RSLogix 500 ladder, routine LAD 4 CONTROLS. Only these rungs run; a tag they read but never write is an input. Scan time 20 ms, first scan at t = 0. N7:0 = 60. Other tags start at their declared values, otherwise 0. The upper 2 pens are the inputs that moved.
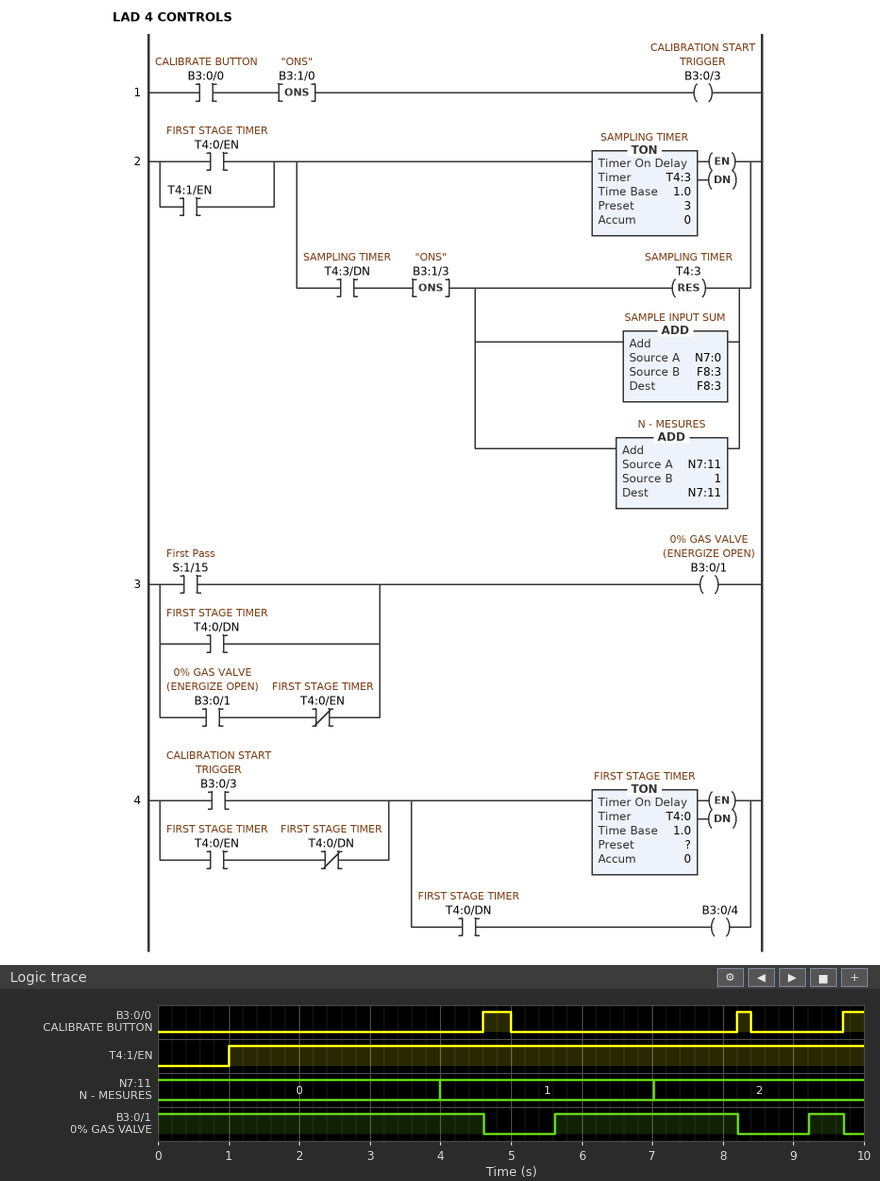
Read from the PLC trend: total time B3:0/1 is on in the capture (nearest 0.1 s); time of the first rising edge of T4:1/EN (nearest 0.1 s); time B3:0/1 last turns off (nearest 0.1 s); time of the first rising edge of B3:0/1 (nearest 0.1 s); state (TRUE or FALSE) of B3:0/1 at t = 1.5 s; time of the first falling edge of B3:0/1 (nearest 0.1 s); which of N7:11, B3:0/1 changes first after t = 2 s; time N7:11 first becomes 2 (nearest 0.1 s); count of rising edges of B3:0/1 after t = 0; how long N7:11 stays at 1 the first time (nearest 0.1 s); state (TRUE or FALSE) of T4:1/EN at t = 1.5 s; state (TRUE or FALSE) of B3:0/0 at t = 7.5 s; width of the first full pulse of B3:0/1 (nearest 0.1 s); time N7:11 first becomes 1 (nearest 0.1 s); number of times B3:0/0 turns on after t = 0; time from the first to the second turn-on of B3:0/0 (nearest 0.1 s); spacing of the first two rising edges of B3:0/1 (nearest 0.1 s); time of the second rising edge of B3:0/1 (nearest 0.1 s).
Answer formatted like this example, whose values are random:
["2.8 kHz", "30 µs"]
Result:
["7.7 s", "1.0 s", "9.7 s", "5.6 s", "TRUE", "4.6 s", "N7:11", "7.0 s", "2", "3.0 s", "TRUE", "FALSE", "2.6 s", "4.0 s", "3", "3.6 s", "3.6 s", "9.2 s"]
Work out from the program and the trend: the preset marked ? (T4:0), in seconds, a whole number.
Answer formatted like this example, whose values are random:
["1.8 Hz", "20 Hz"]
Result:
["1 s"]
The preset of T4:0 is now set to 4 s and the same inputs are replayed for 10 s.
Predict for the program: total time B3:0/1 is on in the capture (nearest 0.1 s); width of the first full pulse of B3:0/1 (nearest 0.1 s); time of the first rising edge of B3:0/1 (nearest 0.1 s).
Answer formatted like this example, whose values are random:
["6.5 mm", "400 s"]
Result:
["5.7 s", "1.1 s", "8.6 s"]
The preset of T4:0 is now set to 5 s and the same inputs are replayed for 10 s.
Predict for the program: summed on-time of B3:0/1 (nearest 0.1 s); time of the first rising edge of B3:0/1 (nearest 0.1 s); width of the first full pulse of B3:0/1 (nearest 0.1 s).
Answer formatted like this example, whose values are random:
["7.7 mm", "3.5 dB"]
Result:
["4.7 s", "9.6 s", "0.1 s"]
